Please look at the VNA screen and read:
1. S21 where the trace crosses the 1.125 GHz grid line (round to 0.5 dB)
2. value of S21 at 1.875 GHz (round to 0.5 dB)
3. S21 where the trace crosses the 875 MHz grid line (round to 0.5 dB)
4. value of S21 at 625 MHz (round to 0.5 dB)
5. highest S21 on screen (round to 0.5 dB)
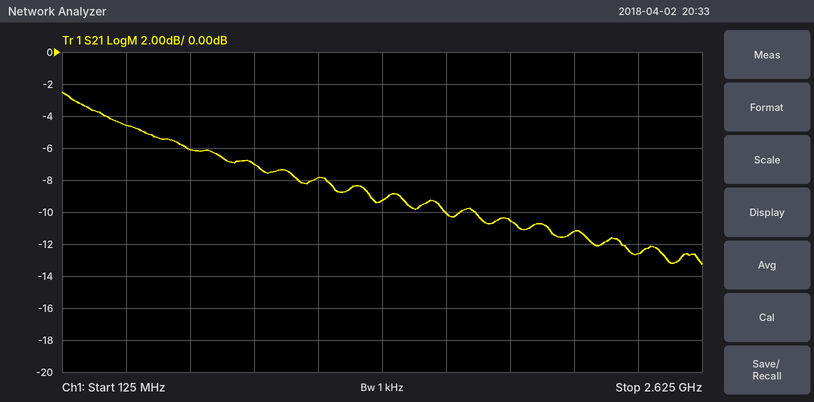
-8.0 dB
-10.5 dB
-7.0 dB
-6.0 dB
-2.5 dB
